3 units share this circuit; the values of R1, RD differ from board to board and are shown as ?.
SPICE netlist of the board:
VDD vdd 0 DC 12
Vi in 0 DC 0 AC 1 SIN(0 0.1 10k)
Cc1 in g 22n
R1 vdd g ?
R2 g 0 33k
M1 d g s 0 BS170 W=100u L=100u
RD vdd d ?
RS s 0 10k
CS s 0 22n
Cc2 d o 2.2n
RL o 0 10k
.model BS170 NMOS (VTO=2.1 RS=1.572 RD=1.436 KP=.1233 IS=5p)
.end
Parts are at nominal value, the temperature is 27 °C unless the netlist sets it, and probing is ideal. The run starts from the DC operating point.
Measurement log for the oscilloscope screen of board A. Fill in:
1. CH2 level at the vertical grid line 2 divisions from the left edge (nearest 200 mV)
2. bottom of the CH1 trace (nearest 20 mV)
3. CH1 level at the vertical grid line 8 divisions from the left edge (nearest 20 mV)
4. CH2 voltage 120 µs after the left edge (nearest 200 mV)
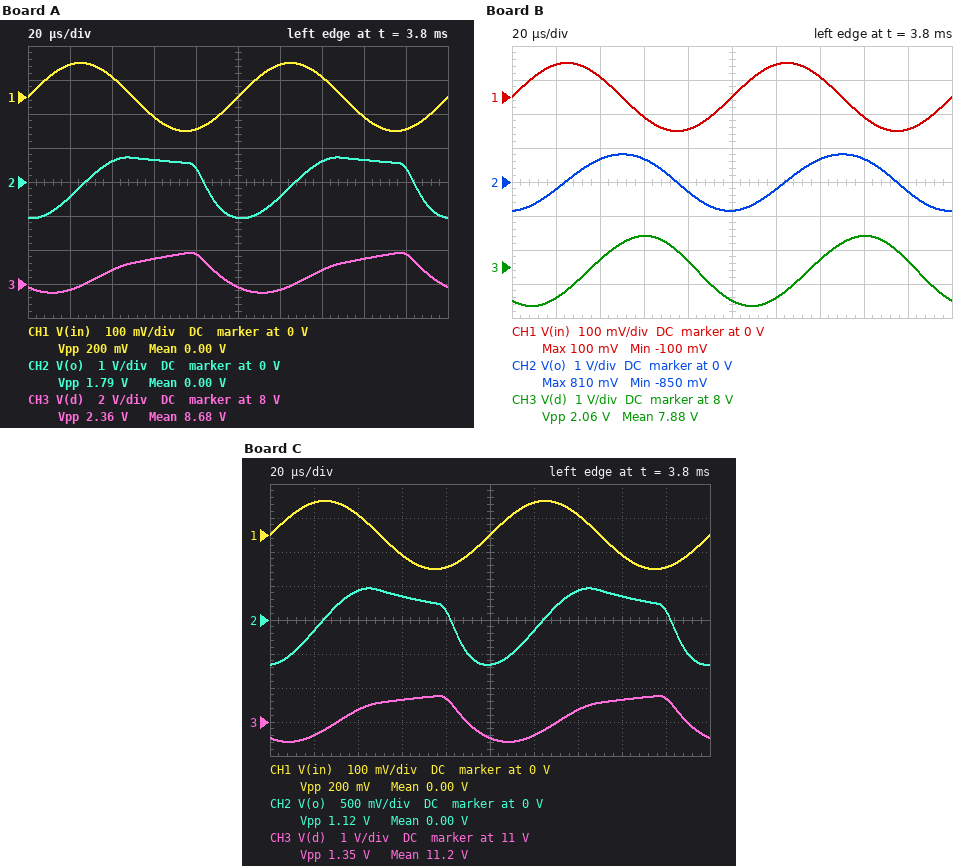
600 mV
-100 mV
-60 mV
-400 mV
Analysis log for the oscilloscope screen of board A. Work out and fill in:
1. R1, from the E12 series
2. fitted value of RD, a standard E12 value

100 kΩ
39 kΩ
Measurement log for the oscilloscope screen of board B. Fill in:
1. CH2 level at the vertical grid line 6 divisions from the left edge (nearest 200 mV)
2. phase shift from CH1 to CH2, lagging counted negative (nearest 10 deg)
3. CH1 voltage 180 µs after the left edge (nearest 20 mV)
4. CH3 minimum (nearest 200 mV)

-200 mV
-90 deg
-100 mV
6.8 V
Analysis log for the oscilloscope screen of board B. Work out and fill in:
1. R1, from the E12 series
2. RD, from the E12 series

56 kΩ
18 kΩ
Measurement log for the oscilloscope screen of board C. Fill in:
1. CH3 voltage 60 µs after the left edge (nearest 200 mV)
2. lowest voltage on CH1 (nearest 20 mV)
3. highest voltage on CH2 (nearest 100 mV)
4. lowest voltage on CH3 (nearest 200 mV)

11.6 V
-100 mV
500 mV
10.4 V
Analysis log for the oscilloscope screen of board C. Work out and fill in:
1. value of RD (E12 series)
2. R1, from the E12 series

10 kΩ
100 kΩ
